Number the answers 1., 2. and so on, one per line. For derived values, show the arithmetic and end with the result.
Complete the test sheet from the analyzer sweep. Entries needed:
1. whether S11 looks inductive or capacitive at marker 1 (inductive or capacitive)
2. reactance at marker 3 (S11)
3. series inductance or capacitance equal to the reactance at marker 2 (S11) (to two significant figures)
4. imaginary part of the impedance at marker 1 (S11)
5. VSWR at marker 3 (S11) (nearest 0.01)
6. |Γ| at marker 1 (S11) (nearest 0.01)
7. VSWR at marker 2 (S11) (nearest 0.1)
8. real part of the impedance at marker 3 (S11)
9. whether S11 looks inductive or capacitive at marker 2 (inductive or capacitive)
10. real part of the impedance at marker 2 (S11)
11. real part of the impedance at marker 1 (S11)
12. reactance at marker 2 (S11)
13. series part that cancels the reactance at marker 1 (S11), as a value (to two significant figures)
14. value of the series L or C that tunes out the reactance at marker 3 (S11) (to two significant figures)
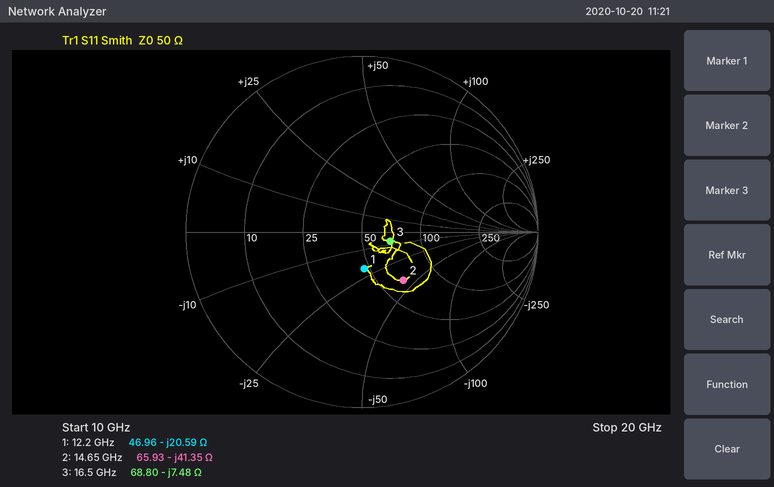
1. capacitive
2. -7.48 Ω
3. C = 1/(2π × 14.65 GHz × 41.35 Ω) ≈ 263 fF, so 260 fF to two significant figures
4. -20.59 Ω
5. 1.41
6. 0.21
7. 2.1
8. 68.80 Ω
9. capacitive
10. 65.93 Ω
11. 46.96 Ω
12. -41.35 Ω
13. L = 20.59 Ω/(2π × 12.2 GHz) ≈ 269 pH, so 270 pH to two significant figures
14. L = 7.48 Ω/(2π × 16.5 GHz) ≈ 72 pH
